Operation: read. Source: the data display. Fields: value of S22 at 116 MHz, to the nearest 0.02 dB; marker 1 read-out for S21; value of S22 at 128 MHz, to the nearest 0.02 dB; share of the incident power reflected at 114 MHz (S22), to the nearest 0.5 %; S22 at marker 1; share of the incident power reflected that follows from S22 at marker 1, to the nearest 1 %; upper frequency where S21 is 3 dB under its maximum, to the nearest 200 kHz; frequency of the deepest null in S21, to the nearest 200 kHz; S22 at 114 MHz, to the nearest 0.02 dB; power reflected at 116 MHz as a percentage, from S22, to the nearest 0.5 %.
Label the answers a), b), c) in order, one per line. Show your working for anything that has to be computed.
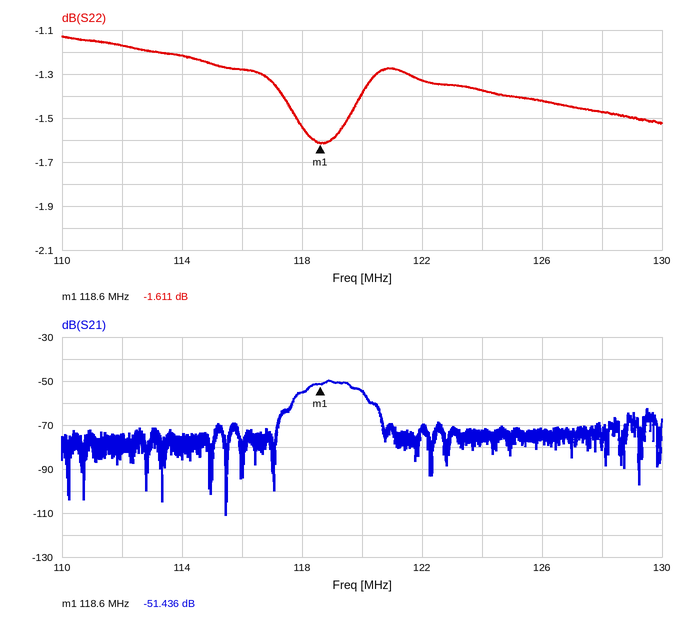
a) -1.28 dB
b) -51.436 dB
c) -1.48 dB
d) 10^(-1.22/10) ≈ 75.5 %
e) -1.611 dB
f) 10^(-1.611/10) ≈ 69 %
g) 119.6 MHz
h) 115.4 MHz
i) -1.22 dB
j) 10^(-1.28/10) ≈ 74.5 %
